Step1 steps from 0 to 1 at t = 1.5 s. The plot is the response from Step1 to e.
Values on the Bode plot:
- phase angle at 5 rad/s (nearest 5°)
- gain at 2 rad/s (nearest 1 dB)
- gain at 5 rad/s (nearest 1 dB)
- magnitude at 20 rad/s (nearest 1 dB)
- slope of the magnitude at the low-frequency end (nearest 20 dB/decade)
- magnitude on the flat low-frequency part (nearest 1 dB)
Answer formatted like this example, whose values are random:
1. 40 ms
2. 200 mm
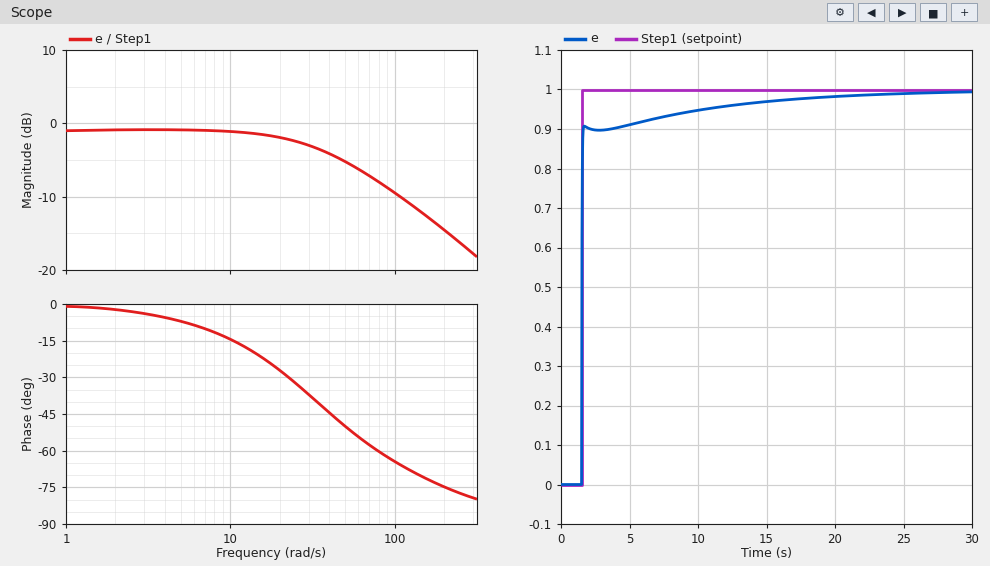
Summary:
1. -5°
2. -1 dB
3. -1 dB
4. -2 dB
5. 0 dB/decade
6. -1 dB
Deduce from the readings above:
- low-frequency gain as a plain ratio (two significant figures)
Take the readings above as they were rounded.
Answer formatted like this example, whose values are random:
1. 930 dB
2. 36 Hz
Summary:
1. 0.89
